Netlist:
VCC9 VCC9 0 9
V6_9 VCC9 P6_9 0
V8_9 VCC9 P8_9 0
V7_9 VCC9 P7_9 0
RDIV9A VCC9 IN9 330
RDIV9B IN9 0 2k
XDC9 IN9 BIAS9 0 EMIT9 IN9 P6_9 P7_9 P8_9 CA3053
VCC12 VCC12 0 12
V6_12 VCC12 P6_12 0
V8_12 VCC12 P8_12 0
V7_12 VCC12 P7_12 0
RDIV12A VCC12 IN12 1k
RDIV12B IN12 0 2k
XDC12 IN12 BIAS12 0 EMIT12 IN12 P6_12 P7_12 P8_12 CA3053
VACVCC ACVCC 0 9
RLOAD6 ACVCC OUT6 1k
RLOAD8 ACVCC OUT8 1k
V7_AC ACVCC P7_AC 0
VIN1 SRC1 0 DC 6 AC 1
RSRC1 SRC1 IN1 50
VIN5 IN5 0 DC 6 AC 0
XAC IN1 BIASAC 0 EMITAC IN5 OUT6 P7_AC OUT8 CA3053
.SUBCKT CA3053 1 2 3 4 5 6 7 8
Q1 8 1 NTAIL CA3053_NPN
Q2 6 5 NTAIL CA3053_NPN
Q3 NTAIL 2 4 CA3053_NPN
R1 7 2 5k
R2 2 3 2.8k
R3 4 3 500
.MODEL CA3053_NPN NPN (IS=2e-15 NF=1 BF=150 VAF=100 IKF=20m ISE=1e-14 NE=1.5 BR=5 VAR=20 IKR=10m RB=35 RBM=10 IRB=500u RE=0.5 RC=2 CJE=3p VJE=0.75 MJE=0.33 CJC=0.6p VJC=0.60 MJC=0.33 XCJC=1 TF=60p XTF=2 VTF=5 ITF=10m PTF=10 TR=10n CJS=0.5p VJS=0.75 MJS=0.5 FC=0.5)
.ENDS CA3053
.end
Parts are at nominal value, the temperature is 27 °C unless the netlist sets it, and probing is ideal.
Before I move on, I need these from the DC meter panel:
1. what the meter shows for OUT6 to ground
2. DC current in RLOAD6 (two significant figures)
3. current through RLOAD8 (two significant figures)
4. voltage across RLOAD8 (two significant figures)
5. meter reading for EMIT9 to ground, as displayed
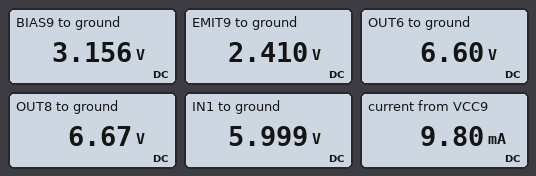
6.60 V
2.4 mA
2.3 mA
2.3 V
2.410 V
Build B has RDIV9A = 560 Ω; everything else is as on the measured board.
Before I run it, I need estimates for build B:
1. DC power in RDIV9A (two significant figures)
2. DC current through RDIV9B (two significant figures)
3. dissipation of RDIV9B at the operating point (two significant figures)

7.0 mW
3.5 mA
25 mW
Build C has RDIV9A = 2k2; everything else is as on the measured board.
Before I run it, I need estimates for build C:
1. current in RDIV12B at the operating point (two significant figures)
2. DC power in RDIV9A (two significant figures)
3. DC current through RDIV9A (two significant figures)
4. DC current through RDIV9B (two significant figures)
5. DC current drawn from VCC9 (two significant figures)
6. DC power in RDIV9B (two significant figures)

4.0 mA
10 mW
2.2 mA
2.1 mA
8.1 mA
9.0 mW
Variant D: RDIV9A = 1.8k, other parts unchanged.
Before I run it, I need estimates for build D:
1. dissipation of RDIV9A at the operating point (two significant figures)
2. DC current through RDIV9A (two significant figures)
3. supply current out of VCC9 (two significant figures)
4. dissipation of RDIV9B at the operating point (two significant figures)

10 mW
2.4 mA
8.3 mA
11 mW
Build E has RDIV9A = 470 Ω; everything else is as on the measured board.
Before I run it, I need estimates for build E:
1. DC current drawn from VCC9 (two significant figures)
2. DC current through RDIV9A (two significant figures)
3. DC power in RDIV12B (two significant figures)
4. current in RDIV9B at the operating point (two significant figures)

9.6 mA
3.7 mA
32 mW
3.6 mA
